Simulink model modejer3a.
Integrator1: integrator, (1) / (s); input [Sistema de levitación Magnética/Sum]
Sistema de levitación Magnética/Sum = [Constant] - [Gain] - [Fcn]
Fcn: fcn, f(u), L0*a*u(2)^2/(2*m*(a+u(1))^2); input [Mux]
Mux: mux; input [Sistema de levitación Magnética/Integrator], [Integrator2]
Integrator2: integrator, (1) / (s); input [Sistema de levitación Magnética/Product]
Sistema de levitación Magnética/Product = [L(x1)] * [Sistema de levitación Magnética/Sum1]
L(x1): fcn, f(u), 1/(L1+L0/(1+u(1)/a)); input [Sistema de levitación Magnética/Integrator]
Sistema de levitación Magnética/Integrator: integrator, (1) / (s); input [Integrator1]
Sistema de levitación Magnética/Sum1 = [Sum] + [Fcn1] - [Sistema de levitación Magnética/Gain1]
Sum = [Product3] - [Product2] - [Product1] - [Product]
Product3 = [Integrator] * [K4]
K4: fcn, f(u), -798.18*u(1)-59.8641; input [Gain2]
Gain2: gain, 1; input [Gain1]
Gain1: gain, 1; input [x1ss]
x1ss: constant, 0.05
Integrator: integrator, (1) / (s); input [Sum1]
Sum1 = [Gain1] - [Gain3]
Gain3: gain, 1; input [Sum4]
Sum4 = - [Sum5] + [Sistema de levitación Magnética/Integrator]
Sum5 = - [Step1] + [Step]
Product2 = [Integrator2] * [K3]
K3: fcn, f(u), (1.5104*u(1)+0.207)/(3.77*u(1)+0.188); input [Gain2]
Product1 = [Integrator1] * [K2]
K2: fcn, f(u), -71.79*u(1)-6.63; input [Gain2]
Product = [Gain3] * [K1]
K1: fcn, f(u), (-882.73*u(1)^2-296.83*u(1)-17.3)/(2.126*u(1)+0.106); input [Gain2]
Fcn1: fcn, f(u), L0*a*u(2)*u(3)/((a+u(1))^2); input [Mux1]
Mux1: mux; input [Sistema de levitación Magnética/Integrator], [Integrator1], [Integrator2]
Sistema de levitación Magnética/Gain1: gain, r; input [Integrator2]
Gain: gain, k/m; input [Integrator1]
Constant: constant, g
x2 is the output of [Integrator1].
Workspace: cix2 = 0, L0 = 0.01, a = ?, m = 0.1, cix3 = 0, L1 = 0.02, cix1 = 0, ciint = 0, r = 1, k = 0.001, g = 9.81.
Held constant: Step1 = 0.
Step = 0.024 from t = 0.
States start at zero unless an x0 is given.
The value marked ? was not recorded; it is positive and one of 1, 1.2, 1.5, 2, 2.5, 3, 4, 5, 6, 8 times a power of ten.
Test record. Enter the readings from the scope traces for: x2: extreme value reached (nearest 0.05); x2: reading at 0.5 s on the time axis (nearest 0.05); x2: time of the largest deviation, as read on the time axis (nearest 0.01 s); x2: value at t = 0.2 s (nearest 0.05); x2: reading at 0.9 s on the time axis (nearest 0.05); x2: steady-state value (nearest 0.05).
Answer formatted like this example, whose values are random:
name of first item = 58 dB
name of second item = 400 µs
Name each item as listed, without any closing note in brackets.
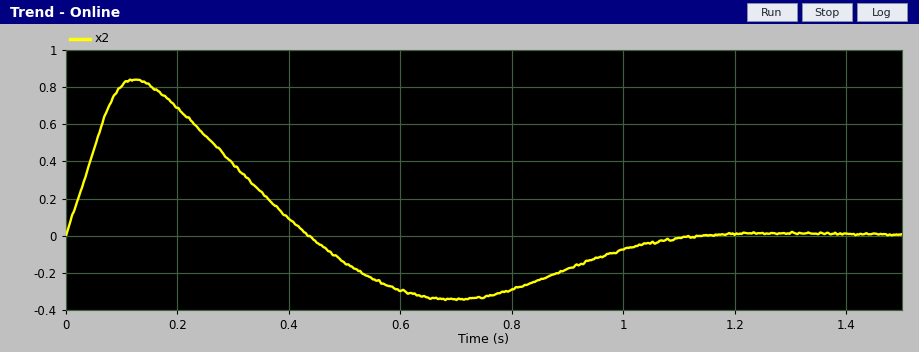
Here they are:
x2: extreme value reached = 0.85
x2: reading at 0.5 s on the time axis = -0.15
x2: time of the largest deviation, as read on the time axis = 0.12 s
x2: value at t = 0.2 s = 0.70
x2: reading at 0.9 s on the time axis = -0.20
x2: steady-state value = 0.00
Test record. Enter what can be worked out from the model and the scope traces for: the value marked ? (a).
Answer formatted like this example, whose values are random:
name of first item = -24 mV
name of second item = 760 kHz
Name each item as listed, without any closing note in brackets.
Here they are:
the value marked ? = 0.05
